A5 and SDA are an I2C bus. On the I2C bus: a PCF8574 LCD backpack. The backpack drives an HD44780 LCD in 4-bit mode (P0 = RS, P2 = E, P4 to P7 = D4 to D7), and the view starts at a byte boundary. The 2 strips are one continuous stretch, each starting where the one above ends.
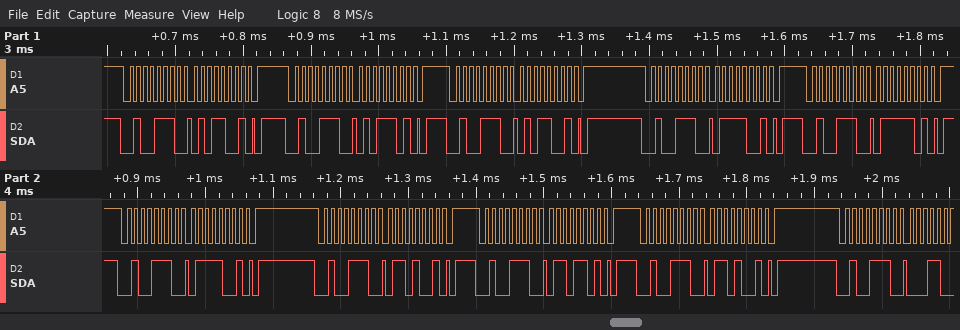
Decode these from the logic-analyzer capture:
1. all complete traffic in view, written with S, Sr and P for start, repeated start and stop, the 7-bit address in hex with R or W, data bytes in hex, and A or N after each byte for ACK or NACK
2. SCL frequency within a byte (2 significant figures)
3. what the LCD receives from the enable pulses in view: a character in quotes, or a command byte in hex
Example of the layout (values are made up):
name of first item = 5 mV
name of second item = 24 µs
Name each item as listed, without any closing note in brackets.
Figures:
all complete traffic in view, written with S, Sr and P for start, repeated start and stop, the 7-bit address in hex with R or W, data bytes in hex, and A or N after each byte for ACK or NACK = S 27W A 59 A P S 27W A 5D A P S 27W A 59 A P S 27W A 79 A P S 27W A 7D A P S 27W A 79 A P S 27W A 69 A P S 27W A 6D A P S 27W A 69 A P S 27W A
SCL frequency within a byte = 100 kHz
what the LCD receives from the enable pulses in view: a character in quotes, or a command byte in hex = 'W'
